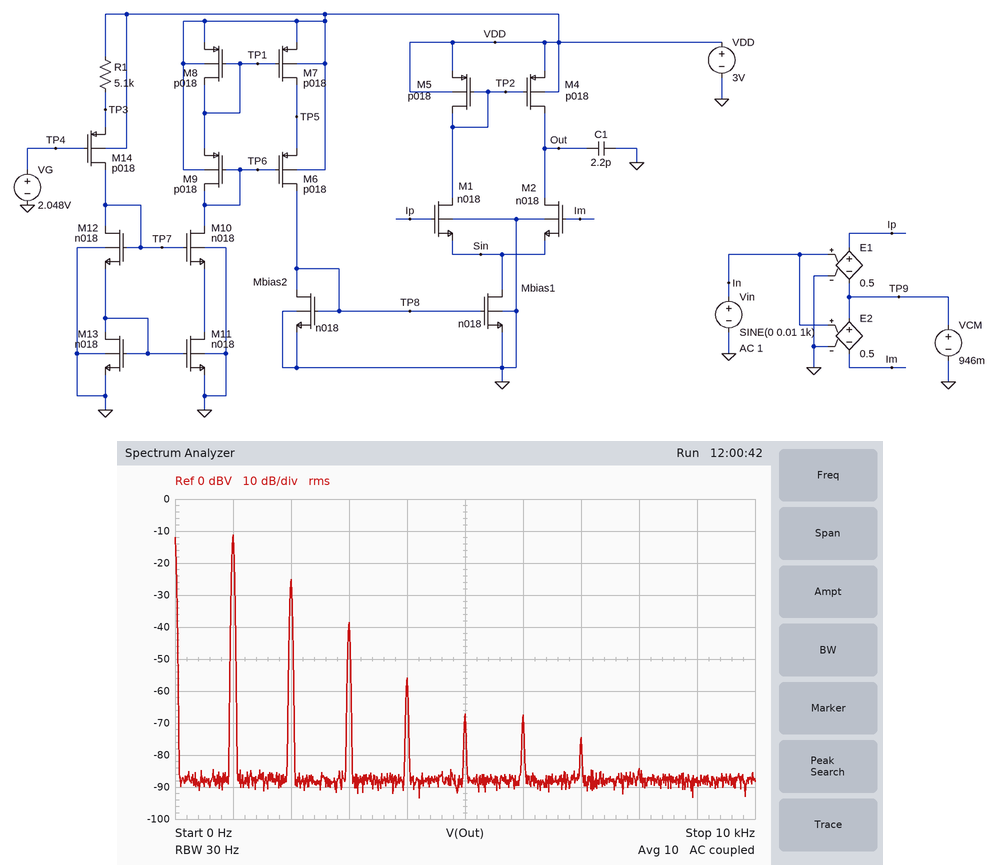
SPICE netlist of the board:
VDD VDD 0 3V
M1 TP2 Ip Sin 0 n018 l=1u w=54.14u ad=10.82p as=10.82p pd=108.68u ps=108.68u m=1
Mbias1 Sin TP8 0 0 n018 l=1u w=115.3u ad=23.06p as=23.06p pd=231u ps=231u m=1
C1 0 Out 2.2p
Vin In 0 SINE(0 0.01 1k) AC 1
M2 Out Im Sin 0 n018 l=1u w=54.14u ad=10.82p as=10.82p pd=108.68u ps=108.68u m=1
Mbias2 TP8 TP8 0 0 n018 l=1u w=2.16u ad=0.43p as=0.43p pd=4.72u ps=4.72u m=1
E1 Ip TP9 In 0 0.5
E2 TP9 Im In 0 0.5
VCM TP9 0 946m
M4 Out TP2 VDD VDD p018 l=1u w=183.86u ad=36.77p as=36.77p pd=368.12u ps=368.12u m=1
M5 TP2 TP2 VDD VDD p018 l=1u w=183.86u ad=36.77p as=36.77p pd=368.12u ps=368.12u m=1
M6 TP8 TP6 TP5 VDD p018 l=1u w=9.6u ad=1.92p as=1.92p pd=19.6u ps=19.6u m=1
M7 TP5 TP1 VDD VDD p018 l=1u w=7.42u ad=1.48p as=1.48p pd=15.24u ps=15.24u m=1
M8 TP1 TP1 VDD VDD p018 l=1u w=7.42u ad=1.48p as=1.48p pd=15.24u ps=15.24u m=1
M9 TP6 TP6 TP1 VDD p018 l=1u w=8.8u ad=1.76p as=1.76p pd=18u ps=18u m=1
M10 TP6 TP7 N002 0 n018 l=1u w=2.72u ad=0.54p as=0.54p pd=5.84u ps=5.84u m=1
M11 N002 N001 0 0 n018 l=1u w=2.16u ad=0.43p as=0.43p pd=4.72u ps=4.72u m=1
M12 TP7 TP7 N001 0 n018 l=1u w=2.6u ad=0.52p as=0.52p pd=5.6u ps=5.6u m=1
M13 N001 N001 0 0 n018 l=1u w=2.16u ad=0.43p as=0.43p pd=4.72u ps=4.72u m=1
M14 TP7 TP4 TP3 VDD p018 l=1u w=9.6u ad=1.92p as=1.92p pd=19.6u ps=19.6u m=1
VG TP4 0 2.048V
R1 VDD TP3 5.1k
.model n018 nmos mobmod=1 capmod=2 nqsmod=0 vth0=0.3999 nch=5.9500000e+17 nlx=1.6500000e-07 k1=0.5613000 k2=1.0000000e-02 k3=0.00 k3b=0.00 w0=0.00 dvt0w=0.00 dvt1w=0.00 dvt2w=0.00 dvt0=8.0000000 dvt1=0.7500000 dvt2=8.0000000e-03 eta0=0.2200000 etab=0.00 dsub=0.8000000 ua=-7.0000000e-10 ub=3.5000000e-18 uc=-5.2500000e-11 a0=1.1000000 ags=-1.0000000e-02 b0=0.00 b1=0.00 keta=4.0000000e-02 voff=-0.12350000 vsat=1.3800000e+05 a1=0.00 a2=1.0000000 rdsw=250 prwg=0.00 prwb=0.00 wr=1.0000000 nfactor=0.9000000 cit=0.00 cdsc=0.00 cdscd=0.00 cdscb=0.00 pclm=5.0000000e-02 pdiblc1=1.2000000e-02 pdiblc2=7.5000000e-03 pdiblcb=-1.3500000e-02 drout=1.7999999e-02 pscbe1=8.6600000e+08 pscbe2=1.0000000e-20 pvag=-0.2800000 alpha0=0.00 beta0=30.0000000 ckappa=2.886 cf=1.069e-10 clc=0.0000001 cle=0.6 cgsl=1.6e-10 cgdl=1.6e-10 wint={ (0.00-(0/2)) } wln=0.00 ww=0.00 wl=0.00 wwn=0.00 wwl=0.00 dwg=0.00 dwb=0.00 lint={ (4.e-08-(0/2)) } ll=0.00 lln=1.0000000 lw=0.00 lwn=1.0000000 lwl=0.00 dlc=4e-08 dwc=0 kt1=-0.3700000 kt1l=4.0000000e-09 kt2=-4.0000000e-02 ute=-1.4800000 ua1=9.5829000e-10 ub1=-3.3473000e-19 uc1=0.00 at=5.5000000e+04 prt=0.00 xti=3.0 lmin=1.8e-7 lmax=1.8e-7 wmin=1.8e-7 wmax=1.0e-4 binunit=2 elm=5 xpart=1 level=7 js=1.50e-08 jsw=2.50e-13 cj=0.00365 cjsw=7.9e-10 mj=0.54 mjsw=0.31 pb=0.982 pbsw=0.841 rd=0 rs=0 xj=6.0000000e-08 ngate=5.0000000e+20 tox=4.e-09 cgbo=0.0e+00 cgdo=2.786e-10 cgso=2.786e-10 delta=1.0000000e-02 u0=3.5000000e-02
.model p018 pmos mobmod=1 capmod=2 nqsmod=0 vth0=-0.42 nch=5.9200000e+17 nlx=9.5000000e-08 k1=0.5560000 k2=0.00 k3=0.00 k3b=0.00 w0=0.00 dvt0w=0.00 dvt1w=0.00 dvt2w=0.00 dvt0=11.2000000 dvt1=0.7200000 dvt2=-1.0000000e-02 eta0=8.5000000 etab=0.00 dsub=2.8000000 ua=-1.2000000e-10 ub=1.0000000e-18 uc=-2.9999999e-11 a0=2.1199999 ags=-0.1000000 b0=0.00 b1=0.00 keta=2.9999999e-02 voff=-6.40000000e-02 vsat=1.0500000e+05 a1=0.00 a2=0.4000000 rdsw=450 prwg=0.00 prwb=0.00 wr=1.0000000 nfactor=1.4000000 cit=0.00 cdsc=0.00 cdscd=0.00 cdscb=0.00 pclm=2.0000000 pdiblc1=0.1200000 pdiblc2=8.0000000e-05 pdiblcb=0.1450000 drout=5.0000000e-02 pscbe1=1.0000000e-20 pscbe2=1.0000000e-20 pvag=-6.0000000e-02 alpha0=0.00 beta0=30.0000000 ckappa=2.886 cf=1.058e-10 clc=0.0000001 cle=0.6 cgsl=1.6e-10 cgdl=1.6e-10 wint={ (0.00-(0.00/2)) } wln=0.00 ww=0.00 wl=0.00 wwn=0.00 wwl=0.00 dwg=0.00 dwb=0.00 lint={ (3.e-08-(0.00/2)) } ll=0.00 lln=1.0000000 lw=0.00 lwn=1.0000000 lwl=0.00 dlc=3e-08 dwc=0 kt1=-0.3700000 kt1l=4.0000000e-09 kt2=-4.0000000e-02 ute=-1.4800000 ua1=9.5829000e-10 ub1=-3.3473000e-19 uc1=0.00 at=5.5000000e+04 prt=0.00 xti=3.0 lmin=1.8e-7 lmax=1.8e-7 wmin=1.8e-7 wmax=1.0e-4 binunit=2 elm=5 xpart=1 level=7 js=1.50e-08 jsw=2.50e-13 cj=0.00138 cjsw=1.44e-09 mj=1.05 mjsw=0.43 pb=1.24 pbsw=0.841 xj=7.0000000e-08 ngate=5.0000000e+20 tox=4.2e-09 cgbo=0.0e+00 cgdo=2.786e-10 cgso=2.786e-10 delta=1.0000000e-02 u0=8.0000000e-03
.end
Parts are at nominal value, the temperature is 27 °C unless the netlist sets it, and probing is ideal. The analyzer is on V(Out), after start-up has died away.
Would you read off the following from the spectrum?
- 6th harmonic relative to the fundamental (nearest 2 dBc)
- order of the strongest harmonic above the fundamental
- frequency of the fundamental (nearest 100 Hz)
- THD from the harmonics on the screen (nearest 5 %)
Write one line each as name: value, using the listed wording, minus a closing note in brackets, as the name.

6th harmonic relative to the fundamental: -56 dBc
order of the strongest harmonic above the fundamental: 2
frequency of the fundamental: 1.0 kHz
THD from the harmonics on the screen: 20 %
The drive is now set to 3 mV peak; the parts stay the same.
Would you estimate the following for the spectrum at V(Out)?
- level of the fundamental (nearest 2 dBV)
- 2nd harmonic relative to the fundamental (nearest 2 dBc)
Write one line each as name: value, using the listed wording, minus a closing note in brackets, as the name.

level of the fundamental: -22 dBV
2nd harmonic relative to the fundamental: -24 dBc
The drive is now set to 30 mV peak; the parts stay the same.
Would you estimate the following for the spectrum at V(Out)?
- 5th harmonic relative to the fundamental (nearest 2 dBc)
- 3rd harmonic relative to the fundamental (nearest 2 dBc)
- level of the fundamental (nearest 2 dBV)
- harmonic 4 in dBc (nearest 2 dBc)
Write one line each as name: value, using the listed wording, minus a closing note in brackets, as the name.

5th harmonic relative to the fundamental: -36 dBc
3rd harmonic relative to the fundamental: -22 dBc
level of the fundamental: -2 dBV
harmonic 4 in dBc: -22 dBc
